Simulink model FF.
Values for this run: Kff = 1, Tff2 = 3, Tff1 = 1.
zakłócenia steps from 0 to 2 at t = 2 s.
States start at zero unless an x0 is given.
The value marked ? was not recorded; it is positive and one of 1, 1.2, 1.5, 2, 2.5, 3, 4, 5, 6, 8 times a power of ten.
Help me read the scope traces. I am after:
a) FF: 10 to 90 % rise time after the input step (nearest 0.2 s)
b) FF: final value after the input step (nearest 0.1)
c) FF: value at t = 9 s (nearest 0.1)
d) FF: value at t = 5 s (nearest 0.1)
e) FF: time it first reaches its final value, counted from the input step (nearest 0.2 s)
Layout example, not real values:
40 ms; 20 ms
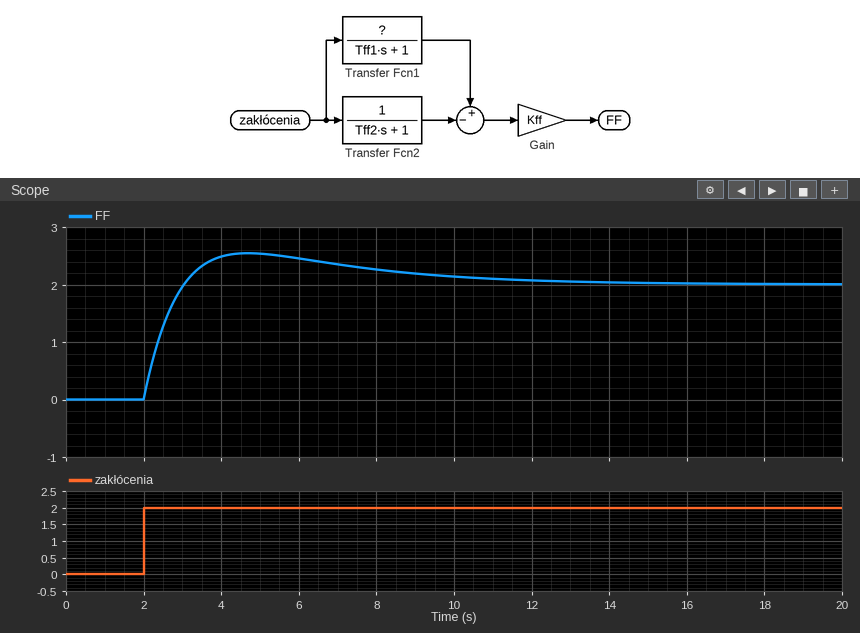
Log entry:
0.8 s; 2.0; 2.2; 2.5; 1.0 s
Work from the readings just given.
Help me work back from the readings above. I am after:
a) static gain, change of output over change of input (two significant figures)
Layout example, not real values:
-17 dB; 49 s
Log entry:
1.0
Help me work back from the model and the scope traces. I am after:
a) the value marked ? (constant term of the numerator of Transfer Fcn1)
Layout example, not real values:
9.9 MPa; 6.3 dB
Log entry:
2
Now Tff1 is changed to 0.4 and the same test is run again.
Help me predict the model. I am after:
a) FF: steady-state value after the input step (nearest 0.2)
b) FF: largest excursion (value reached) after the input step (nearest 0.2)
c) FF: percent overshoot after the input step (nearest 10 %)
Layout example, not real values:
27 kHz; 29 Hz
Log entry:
2.0; 3.2; 60 %
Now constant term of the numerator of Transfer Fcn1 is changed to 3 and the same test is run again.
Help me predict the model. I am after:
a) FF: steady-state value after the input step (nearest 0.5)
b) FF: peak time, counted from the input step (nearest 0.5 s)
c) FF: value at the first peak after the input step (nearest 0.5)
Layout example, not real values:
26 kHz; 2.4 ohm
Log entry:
4.0; 3.5 s; 4.5
